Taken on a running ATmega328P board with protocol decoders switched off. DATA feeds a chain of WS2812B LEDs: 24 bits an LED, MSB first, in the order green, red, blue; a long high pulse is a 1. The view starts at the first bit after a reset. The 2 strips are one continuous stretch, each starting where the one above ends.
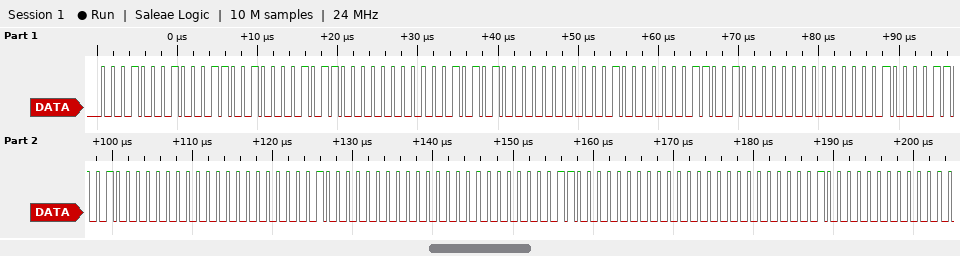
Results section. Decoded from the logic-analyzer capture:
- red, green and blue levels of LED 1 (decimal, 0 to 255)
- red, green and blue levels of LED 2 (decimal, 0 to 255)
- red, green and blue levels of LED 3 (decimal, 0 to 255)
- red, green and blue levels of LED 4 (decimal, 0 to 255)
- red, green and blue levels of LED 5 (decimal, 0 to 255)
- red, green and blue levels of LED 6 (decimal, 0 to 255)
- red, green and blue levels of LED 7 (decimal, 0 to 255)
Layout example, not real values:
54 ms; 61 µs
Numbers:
25, 17, 11; 21, 0, 0; 25, 16, 0; 25, 2, 0; 8, 0, 0; 12, 0, 0; 2, 0, 0
